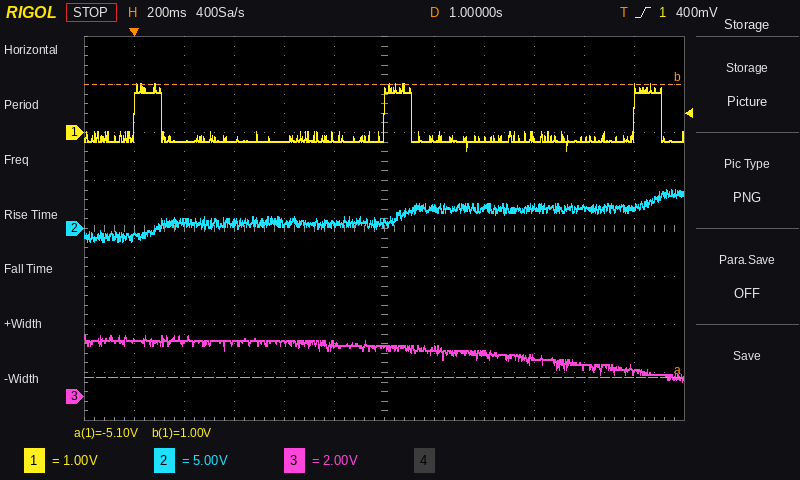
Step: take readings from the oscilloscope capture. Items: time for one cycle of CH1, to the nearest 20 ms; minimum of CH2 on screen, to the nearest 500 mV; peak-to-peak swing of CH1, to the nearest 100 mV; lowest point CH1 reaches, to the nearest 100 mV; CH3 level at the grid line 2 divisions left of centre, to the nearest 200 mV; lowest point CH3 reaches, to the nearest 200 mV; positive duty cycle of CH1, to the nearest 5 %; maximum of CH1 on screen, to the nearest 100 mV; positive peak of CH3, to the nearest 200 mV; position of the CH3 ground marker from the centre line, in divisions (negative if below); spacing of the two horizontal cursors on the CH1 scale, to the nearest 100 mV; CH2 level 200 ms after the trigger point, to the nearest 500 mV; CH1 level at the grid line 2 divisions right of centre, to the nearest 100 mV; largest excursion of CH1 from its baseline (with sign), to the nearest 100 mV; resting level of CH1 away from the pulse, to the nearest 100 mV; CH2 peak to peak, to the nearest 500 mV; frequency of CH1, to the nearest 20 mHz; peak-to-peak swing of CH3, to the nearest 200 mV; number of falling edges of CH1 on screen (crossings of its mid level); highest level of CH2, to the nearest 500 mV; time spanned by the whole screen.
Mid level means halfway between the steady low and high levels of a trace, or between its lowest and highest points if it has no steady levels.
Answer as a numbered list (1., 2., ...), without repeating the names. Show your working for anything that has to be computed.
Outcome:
1. 1.00 s
2. -1.5 V
3. 1.0 V − (-400 mV) = 1.4 V
4. -400 mV
5. 2.2 V
6. 600 mV
7. 10 %
8. 1.0 V
9. 2.6 V
10. -3.5 div
11. 6.1 V
12. 500 mV
13. -100 mV
14. 1.0 V − (-200 mV) = +1.2 V
15. -200 mV
16. 4.0 V − (-1.5 V) = 5.5 V
17. 1 / 1.00 s ≈ 1.00 Hz
18. 2.6 V − (600 mV) = 2.0 V
19. 3
20. 4.0 V
21. 2.4 s
